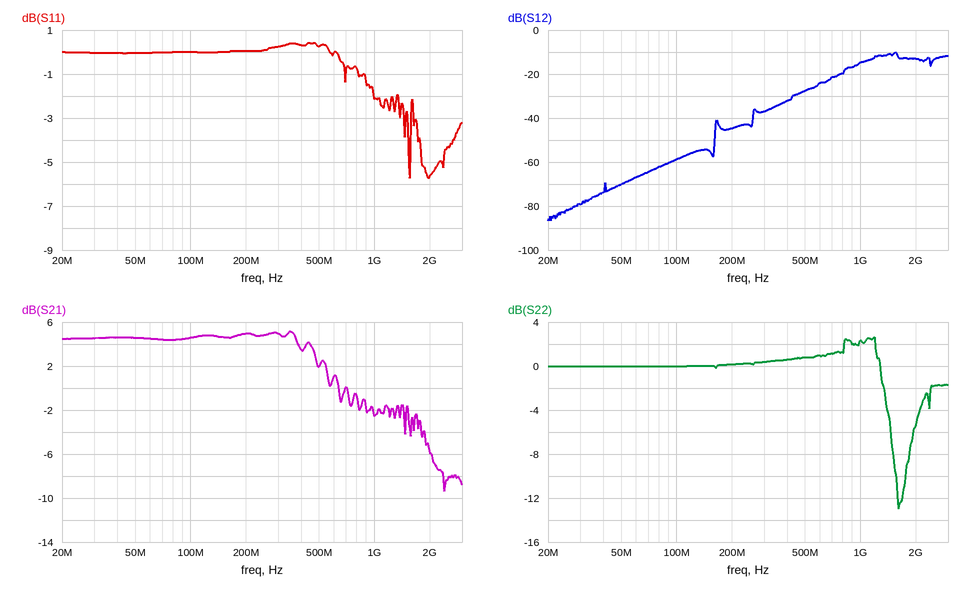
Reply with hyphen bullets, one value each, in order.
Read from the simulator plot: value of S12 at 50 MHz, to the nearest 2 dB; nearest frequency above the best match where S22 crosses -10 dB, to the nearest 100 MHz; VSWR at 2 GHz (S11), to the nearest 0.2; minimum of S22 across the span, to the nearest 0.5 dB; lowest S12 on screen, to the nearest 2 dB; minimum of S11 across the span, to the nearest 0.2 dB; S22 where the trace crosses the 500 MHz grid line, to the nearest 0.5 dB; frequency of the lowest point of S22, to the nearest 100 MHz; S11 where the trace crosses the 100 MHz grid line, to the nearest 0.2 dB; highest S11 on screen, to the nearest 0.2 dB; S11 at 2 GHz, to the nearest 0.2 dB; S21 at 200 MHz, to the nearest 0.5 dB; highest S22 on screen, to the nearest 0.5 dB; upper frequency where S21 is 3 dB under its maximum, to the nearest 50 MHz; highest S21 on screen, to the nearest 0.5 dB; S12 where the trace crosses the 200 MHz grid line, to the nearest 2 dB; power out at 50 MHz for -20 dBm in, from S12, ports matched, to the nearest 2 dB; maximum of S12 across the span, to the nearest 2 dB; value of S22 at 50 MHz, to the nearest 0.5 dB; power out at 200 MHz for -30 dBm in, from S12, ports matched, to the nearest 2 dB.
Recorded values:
- -70 dB
- 1.8 GHz
- 3.2
- -13.0 dB
- -86 dB
- -5.8 dB
- 1.0 dB
- 1.6 GHz
- 0.0 dB
- 0.4 dB
- -5.6 dB
- 5.0 dB
- 2.5 dB
- 500 MHz
- 5.0 dB
- -44 dB
- -90 dBm
- -10 dB
- 0.0 dB
- -74 dBm
